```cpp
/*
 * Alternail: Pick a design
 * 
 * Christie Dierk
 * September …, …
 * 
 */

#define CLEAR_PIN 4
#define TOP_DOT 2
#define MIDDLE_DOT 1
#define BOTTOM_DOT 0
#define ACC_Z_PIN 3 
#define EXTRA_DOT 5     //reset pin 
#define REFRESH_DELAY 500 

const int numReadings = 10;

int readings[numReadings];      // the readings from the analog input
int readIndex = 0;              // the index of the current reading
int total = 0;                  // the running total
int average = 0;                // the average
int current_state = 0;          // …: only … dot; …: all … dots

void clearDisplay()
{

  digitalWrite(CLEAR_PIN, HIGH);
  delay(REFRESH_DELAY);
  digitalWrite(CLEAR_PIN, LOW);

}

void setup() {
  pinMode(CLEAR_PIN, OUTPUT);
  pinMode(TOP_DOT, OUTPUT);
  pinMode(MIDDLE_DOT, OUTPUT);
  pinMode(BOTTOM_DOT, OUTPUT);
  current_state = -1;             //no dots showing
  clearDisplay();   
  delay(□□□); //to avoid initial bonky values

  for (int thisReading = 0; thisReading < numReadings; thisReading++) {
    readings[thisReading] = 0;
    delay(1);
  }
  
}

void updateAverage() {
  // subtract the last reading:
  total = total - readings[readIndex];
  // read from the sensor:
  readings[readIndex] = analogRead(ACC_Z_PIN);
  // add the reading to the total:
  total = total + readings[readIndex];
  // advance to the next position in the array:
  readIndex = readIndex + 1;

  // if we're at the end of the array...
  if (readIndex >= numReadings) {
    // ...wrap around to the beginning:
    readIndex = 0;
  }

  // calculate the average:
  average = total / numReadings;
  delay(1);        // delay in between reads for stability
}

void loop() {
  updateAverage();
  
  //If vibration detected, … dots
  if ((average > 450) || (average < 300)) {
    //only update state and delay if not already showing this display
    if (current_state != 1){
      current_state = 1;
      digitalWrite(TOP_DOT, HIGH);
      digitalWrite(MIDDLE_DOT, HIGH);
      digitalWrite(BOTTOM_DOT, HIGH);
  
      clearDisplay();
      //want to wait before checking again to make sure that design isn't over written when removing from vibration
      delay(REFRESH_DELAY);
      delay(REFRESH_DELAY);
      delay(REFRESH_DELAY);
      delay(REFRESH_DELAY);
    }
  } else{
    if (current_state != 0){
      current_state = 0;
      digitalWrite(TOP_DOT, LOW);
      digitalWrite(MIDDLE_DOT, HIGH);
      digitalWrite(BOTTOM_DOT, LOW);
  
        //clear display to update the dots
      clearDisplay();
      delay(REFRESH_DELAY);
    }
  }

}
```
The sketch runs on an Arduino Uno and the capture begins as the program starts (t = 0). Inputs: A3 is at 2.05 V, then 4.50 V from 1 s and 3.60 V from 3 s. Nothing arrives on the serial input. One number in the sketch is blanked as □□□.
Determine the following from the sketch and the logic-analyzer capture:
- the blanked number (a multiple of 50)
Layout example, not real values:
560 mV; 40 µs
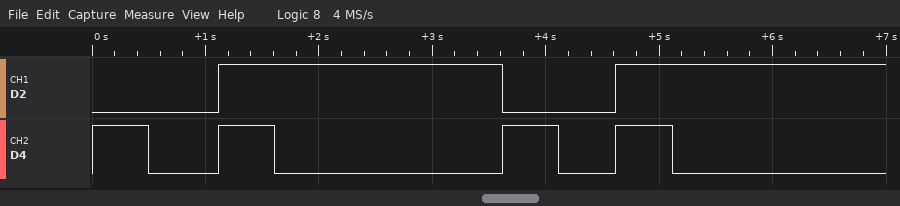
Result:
600
